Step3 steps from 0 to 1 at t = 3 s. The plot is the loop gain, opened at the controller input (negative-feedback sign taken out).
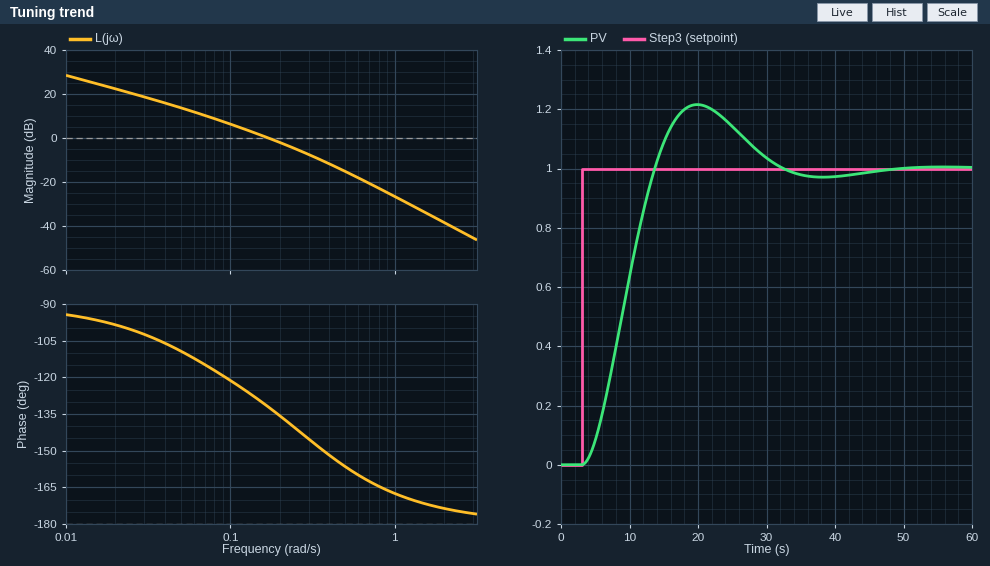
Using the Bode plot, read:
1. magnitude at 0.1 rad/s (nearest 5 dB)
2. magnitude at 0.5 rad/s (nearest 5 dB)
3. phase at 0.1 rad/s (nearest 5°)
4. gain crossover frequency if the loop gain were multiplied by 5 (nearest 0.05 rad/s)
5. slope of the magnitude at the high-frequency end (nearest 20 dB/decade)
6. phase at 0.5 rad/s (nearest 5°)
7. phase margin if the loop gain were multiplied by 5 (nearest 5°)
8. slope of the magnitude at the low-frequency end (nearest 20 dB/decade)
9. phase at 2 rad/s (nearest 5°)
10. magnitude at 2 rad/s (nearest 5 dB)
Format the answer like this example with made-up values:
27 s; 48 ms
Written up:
5 dB; -15 dB; -120°; 0.45 rad/s; -40 dB/decade; -155°; 25°; -20 dB/decade; -175°; -40 dB
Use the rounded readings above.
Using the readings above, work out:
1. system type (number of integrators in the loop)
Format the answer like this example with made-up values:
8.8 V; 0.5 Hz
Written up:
1
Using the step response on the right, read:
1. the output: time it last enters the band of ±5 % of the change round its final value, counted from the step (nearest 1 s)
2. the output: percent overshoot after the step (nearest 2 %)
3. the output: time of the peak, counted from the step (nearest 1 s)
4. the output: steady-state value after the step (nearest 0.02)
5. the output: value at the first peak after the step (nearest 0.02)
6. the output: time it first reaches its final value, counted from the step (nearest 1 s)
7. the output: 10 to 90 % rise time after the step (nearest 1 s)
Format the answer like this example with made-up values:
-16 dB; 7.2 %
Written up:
26 s; 22 %; 17 s; 1.00; 1.22; 11 s; 7 s
